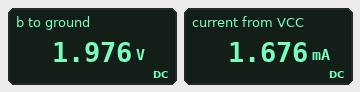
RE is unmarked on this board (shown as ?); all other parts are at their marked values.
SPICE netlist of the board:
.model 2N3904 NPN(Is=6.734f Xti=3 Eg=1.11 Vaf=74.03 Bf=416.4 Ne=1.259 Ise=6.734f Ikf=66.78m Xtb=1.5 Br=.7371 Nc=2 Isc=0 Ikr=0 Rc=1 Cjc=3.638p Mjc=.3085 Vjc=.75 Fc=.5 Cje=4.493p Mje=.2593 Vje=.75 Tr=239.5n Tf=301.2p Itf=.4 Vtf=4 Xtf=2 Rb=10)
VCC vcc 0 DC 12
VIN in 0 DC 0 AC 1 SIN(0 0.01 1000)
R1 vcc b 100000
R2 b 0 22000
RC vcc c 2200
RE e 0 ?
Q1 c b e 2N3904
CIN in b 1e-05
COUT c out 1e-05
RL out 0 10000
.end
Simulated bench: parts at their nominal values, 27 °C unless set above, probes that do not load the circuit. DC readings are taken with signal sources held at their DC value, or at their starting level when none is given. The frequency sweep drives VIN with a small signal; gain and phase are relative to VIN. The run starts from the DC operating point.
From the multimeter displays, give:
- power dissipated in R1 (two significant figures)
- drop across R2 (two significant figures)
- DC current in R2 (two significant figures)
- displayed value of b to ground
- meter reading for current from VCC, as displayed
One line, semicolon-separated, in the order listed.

1.0 mW; 2.0 V; 90 µA; 1.976 V; 1.676 mA
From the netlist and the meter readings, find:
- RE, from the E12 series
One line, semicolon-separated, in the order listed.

820 Ω
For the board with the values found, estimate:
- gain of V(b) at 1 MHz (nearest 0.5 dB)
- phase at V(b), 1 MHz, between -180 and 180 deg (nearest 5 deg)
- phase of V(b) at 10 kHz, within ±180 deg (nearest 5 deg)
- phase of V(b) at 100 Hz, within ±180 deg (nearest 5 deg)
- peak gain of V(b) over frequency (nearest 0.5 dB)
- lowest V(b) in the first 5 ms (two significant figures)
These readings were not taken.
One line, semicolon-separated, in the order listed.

0 dB; 0 deg; 0 deg; 0 deg; 0 dB; 2.0 V
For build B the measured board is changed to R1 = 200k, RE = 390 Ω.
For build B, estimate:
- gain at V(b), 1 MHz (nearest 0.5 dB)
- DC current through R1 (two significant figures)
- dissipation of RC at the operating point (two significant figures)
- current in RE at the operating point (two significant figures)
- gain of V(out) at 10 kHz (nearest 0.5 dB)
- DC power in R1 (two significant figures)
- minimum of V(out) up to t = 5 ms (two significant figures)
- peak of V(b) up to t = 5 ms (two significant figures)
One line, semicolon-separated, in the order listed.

0 dB; 55 µA; 2.2 mW; 1.0 mA; 12.5 dB; 600 µW; -43 mV; 1.1 V
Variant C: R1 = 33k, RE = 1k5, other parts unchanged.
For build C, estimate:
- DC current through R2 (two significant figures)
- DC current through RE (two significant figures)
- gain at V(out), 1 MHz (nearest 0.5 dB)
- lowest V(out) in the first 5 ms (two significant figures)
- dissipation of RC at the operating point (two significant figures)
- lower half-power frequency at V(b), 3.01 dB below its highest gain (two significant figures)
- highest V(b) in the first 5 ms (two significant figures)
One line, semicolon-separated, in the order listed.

210 µA; 2.6 mA; 1.5 dB; -12 mV; 15 mW; 1.3 Hz; 4.6 V
